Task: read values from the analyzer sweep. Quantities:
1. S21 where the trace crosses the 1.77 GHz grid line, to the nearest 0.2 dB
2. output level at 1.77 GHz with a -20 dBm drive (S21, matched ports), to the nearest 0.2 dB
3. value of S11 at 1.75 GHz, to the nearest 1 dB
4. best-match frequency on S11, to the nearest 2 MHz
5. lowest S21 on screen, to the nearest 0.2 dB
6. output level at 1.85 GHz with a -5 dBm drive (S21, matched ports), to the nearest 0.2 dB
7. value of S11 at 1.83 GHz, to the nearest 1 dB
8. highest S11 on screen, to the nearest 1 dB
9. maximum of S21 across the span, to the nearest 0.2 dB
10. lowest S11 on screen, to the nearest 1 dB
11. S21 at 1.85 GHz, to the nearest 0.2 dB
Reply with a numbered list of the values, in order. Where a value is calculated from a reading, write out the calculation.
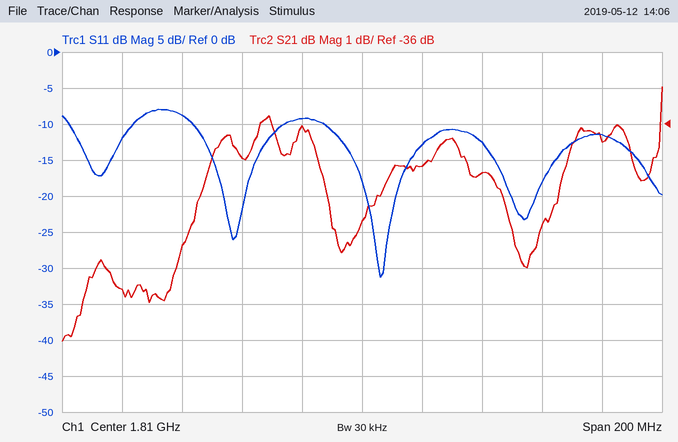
1. -37.0 dB
2. -20 dBm + (-37.0 dB) = -57.0 dBm
3. -9 dB
4. 1.816 GHz
5. -42.0 dB
6. -5 dBm + (-37.4 dB) = -42.4 dBm
7. -13 dB
8. -8 dB
9. -35.0 dB
10. -31 dB
11. -37.4 dB
